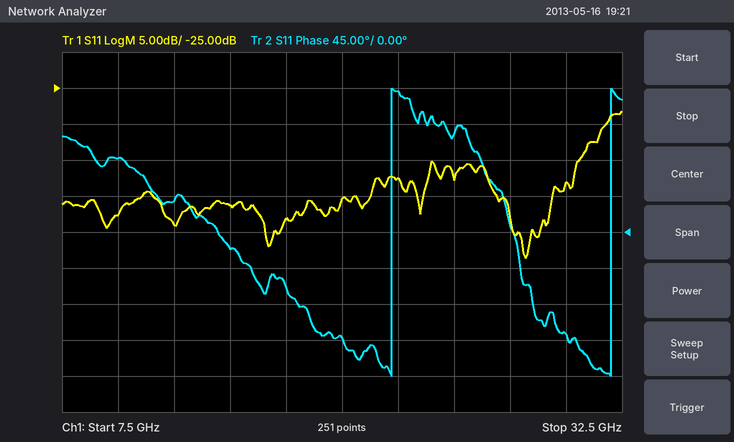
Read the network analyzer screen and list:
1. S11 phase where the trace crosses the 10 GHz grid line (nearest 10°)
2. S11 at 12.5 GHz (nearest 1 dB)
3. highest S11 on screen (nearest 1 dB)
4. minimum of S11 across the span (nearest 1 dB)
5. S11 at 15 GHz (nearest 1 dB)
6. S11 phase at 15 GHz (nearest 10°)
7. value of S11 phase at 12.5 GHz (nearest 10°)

90°
-44 dB
-28 dB
-49 dB
-41 dB
-20°
40°
